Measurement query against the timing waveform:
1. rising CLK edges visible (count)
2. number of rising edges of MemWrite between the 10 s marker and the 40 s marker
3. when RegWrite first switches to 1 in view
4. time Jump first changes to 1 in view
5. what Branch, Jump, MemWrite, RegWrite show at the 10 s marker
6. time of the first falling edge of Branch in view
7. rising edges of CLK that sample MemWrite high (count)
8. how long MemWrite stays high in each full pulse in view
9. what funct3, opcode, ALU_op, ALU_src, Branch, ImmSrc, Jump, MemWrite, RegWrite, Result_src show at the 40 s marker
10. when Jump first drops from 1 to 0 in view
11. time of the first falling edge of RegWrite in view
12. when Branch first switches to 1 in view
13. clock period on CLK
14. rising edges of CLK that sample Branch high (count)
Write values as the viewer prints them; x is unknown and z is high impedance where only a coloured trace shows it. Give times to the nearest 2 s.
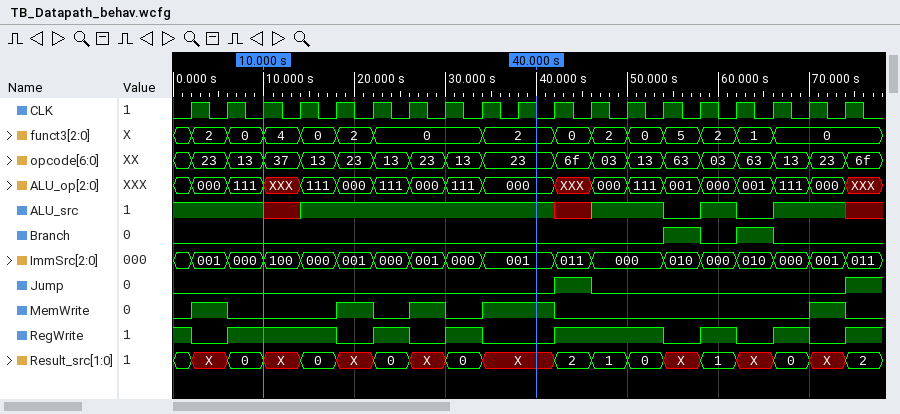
19
3
6 s
42 s
Branch=0, Jump=0, MemWrite=0, RegWrite=1
58 s
6
4 s, 4 s, 4 s, 8 s, 4 s
funct3=2, opcode=23, ALU_op=000, ALU_src=1, Branch=0, ImmSrc=001, Jump=0, MemWrite=1, RegWrite=0, Result_src=X
46 s
2 s
54 s
4 s
2
